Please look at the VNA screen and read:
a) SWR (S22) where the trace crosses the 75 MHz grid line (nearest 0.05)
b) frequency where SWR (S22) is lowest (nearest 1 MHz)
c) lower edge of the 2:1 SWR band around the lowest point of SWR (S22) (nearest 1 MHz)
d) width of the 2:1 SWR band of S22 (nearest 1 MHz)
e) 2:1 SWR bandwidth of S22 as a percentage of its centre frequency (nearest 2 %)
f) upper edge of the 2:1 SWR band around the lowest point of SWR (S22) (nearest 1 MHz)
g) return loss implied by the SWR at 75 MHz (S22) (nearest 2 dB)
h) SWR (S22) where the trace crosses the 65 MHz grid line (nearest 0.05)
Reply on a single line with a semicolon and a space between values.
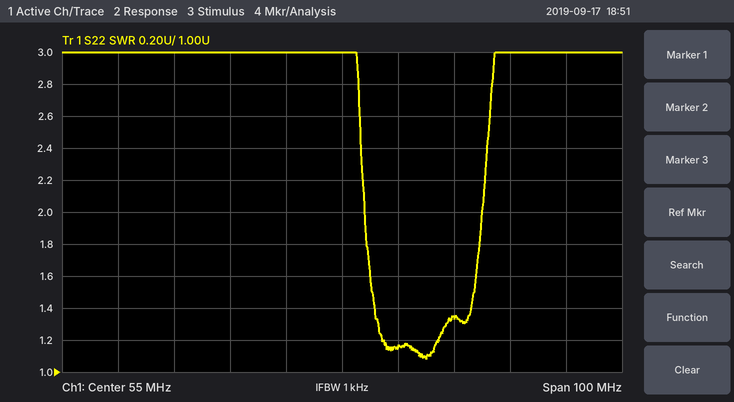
1.35; 70 MHz; 59 MHz; 21 MHz; 30 %; 80 MHz; 16 dB; 1.15
